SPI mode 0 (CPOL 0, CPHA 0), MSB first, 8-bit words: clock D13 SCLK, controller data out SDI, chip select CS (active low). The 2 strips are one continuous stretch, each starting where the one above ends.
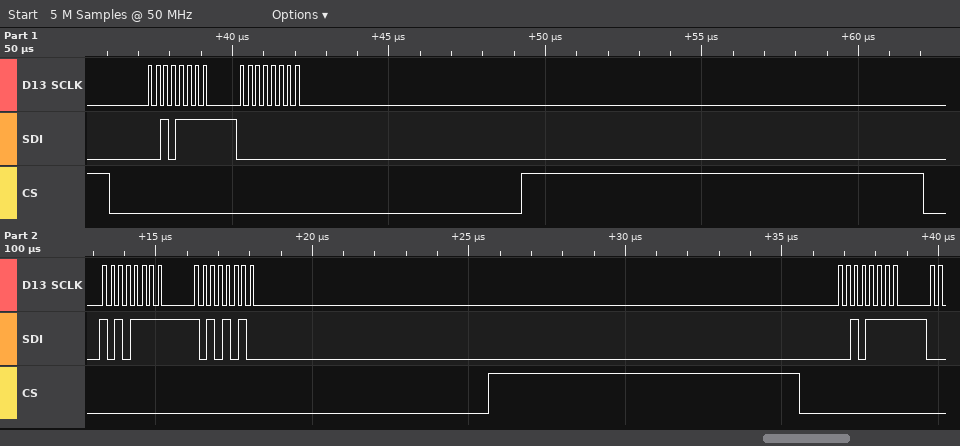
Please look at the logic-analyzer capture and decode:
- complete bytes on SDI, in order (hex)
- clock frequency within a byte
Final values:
2F 00 AF AA 2F
4 MHz
